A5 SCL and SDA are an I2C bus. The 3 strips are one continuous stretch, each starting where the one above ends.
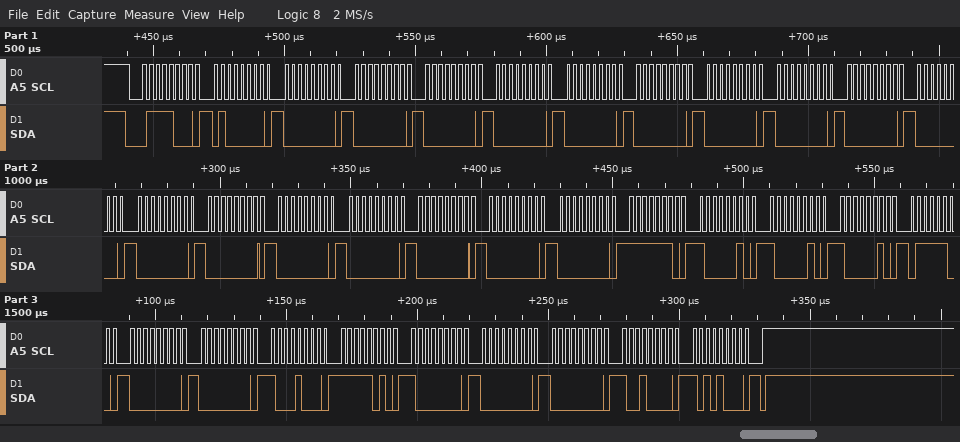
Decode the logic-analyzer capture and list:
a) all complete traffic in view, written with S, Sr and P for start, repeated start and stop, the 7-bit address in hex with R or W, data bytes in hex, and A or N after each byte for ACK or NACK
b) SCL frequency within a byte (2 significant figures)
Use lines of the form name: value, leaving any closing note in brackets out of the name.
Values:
all complete traffic in view, written with S, Sr and P for start, repeated start and stop, the 7-bit address in hex with R or W, data bytes in hex, and A or N after each byte for ACK or NACK: S 3CW A 40 A 00 A 00 A 00 A 00 A 00 A 00 A 00 A 00 A 00 A 00 A 00 A 00 A 00 A 00 A 00 A 00 A 00 A FE A 82 A 82 A 82 A 7C A 00 A 00 A 88 A FA A 80 A 00 A 00 A 90 A A8 A P
SCL frequency within a byte: 400 kHz
